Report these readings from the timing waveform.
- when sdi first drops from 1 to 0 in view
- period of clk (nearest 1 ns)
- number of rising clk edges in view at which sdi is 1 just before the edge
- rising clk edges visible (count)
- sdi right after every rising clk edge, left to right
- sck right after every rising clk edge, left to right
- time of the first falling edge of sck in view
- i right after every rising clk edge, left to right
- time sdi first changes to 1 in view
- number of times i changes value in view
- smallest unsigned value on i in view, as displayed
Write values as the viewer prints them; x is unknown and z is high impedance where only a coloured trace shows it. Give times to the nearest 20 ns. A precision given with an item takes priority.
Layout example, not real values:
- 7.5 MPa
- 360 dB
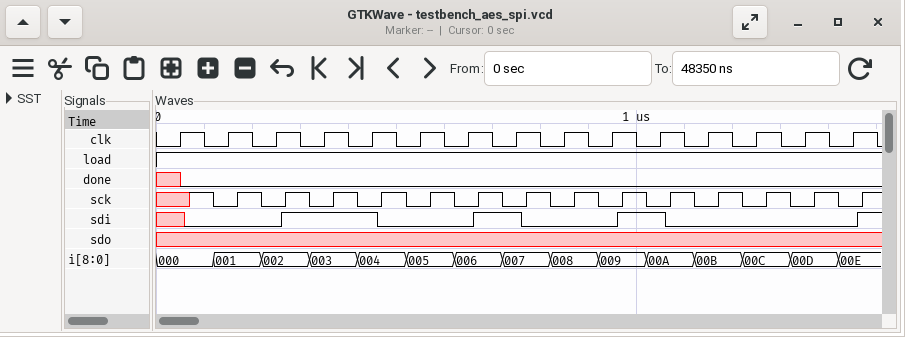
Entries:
- 460 ns
- 100 ns
- 4
- 15
- x 0 0 1 1 0 0 1 0 0 1 0 0 0 0
- x 0 0 0 0 0 0 0 0 0 0 0 0 0 0
- 120 ns
- 000, 001, 002, 003, 004, 005, 006, 007, 008, 009, 00A, 00B, 00C, 00D, 00E
- 260 ns
- 14
- 000
